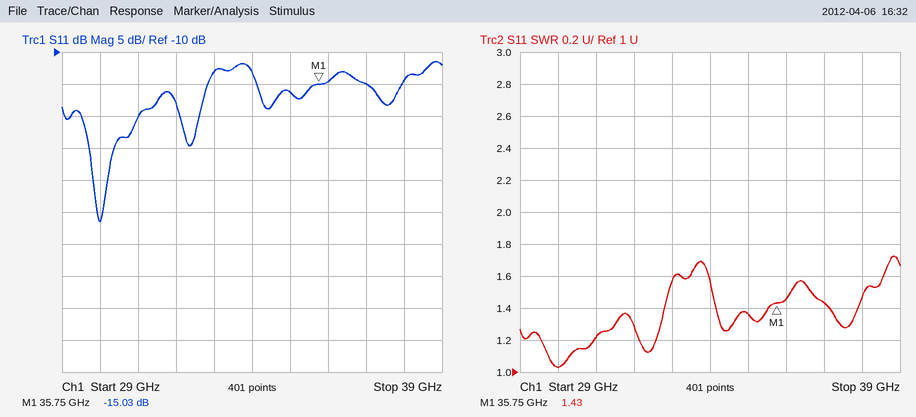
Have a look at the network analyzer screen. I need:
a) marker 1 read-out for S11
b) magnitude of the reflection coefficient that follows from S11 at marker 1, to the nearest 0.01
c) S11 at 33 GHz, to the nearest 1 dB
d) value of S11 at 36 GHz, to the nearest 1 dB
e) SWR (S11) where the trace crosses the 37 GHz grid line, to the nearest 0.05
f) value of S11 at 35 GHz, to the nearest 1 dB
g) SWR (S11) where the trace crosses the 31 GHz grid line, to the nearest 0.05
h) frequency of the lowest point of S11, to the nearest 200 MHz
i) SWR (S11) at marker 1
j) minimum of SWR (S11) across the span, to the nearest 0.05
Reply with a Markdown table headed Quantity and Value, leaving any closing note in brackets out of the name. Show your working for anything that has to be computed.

| Quantity | Value |
|---|---|
| marker 1 read-out for S11 | -15.03 dB |
| magnitude of the reflection coefficient that follows from S11 at marker 1, to the nearest 0.01 | 10^(-15.03/20) ≈ 0.18 |
| S11 at 33 GHz, to the nearest 1 dB | -13 dB |
| value of S11 at 36 GHz, to the nearest 1 dB | -15 dB |
| SWR (S11) where the trace crosses the 37 GHz grid line, to the nearest 0.05 | 1.45 |
| value of S11 at 35 GHz, to the nearest 1 dB | -16 dB |
| SWR (S11) where the trace crosses the 31 GHz grid line, to the nearest 0.05 | 1.20 |
| frequency of the lowest point of S11, to the nearest 200 MHz | 30.0 GHz |
| SWR (S11) at marker 1 | 1.43 |
| minimum of SWR (S11) across the span, to the nearest 0.05 | 1.05 |
